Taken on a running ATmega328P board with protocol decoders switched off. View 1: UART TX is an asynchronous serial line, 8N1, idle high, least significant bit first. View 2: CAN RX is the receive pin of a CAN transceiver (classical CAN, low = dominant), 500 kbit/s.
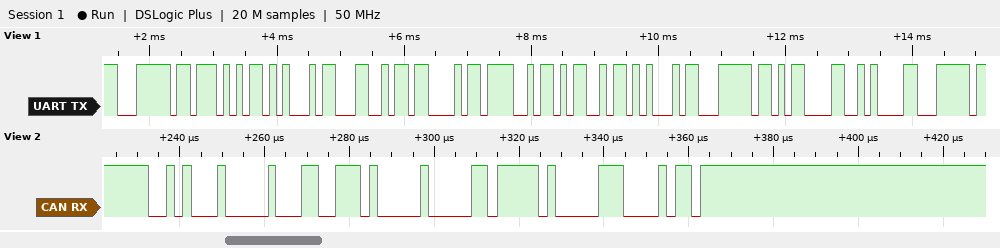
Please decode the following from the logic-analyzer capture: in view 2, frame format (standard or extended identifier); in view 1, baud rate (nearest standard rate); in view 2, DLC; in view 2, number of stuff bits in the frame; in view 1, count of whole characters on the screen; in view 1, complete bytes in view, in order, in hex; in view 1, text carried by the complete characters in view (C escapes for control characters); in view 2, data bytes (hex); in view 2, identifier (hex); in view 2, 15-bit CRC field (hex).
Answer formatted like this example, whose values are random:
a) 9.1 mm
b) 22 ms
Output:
a) standard
b) 9600 baud
c) 3
d) 5
e) 12
f) 0x7C 0x57 0x45 0x4C 0x43 0x4F 0x4D 0x45 0x7C 0x0D 0x0A 0x7C
g) "|WELCOME|\r\n|"
h) 3A 00 5F
i) 0x288
j) 0x4185
